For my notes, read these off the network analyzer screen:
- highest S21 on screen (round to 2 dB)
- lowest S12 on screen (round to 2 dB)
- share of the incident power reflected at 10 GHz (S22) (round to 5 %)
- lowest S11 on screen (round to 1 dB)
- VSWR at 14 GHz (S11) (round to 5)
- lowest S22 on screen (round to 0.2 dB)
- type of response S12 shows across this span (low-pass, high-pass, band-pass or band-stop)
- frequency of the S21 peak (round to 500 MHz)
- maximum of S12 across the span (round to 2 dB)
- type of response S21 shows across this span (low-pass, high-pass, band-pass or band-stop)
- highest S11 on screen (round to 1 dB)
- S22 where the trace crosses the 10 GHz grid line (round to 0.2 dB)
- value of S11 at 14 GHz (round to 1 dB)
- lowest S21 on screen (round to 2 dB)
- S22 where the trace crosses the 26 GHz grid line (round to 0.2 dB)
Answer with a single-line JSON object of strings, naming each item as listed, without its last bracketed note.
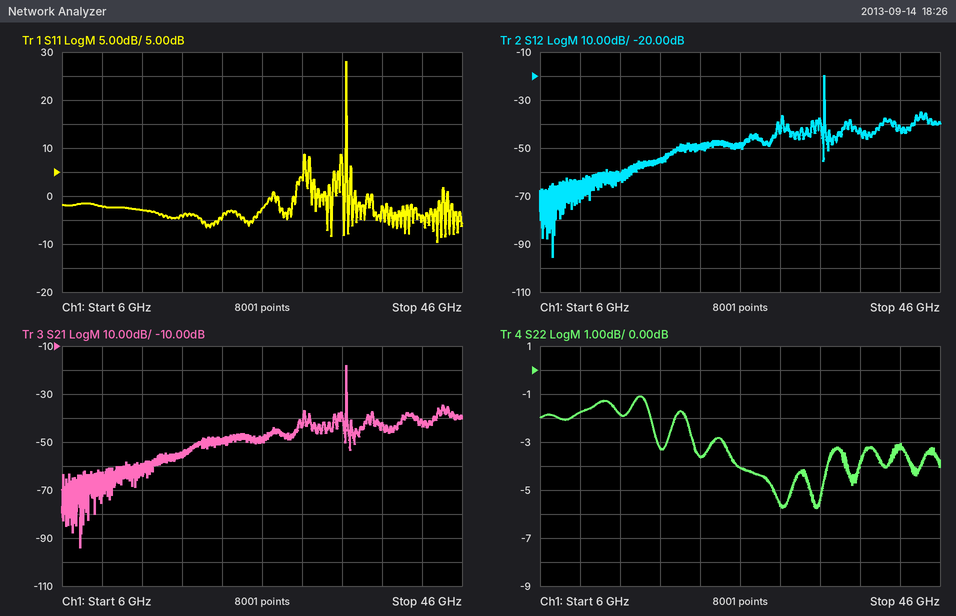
{"highest S21 on screen": "-18 dB", "lowest S12 on screen": "-96 dB", "share of the incident power reflected at 10 GHz (S22)": "65 %", "lowest S11 on screen": "-10 dB", "VSWR at 14 GHz (S11)": "5", "lowest S22 on screen": "-5.8 dB", "type of response S12 shows across this span": "band-pass", "frequency of the S21 peak": "34.5 GHz", "maximum of S12 across the span": "-20 dB", "type of response S21 shows across this span": "band-pass", "highest S11 on screen": "28 dB", "S22 where the trace crosses the 10 GHz grid line": "-1.8 dB", "value of S11 at 14 GHz": "-3 dB", "lowest S21 on screen": "-94 dB", "S22 where the trace crosses the 26 GHz grid line": "-4.0 dB"}
